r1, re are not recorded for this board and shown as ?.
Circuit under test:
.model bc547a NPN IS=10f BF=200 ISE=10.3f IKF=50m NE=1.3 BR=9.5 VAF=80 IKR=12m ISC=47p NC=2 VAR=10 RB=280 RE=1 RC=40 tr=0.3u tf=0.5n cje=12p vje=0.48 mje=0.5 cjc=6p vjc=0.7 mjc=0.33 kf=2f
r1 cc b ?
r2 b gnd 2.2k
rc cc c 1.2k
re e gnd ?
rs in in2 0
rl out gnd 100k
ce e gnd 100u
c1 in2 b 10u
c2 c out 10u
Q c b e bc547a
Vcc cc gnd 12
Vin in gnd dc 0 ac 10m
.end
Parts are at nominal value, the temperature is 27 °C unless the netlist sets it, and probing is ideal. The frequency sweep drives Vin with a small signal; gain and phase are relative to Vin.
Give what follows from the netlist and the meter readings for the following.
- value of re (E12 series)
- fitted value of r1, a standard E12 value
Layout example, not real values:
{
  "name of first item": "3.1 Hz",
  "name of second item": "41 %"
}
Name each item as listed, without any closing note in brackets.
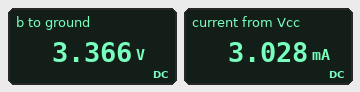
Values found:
{
  "value of re": "1.8 kΩ",
  "fitted value of r1, a standard E12 value": "5.6 kΩ"
}
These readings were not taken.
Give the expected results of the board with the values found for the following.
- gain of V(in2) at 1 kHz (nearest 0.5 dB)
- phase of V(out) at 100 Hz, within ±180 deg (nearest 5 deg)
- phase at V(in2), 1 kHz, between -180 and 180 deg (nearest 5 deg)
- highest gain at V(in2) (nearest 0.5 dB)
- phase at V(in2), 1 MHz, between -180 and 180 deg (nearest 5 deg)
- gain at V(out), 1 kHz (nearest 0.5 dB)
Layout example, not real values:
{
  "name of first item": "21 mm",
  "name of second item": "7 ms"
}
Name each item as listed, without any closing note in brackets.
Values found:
{
  "gain of V(in2) at 1 kHz": "0 dB",
  "phase of V(out) at 100 Hz, within ±180 deg": "-135 deg",
  "phase at V(in2), 1 kHz, between -180 and 180 deg": "0 deg",
  "highest gain at V(in2)": "0 dB",
  "phase at V(in2), 1 MHz, between -180 and 180 deg": "0 deg",
  "gain at V(out), 1 kHz": "35.0 dB"
}
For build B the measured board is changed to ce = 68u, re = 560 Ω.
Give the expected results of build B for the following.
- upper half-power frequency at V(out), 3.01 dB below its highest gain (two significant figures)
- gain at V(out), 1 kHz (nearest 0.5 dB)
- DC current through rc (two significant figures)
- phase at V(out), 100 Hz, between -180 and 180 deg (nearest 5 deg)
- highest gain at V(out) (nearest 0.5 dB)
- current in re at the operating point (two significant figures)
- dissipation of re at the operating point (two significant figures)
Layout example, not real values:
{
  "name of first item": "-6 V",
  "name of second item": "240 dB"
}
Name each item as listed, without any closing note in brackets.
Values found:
{
  "upper half-power frequency at V(out), 3.01 dB below its highest gain": "1.1 MHz",
  "gain at V(out), 1 kHz": "41.0 dB",
  "DC current through rc": "4.6 mA",
  "phase at V(out), 100 Hz, between -180 and 180 deg": "-110 deg",
  "highest gain at V(out)": "41.5 dB",
  "current in re at the operating point": "4.7 mA",
  "dissipation of re at the operating point": "12 mW"
}
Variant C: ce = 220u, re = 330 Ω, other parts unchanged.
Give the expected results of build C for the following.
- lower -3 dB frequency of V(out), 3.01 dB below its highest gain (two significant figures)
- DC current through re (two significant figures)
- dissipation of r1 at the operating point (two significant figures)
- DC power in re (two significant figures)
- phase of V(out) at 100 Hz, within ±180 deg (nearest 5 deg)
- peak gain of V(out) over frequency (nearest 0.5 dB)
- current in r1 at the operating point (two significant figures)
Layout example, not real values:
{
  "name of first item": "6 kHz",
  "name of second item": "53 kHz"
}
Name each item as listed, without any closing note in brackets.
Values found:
{
  "lower -3 dB frequency of V(out), 3.01 dB below its highest gain": "64 Hz",
  "DC current through re": "7.6 mA",
  "dissipation of r1 at the operating point": "14 mW",
  "DC power in re": "19 mW",
  "phase of V(out) at 100 Hz, within ±180 deg": "-145 deg",
  "peak gain of V(out) over frequency": "15.5 dB",
  "current in r1 at the operating point": "1.6 mA"
}
